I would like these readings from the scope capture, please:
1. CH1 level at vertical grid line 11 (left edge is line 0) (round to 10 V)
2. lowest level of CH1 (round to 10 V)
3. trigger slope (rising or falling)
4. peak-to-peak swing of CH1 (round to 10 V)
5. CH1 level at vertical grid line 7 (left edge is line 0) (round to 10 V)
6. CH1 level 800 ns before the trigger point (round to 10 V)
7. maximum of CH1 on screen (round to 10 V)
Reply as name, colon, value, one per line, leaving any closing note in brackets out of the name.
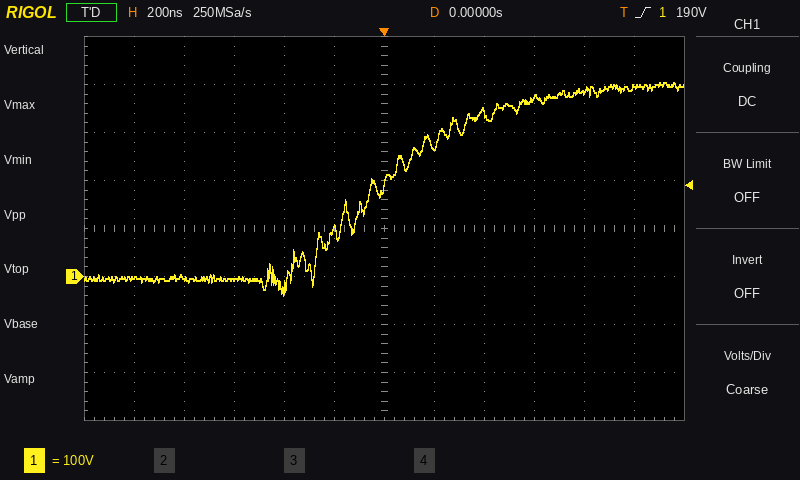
CH1 level at vertical grid line 11 (left edge is line 0): 390 V
lowest level of CH1: -40 V
trigger slope: rising
peak-to-peak swing of CH1: 440 V
CH1 level at vertical grid line 7 (left edge is line 0): 270 V
CH1 level 800 ns before the trigger point: 0 V
maximum of CH1 on screen: 400 V
